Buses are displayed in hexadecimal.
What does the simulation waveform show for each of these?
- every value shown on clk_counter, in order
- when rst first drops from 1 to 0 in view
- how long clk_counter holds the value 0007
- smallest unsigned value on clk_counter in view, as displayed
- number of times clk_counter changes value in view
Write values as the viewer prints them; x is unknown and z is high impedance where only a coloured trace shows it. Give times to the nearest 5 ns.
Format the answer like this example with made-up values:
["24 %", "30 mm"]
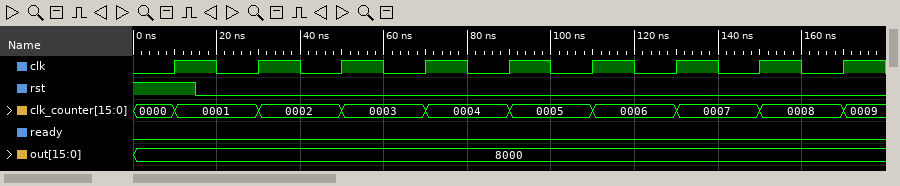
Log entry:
["0000, 0001, 0002, 0003, 0004, 0005, 0006, 0007, 0008, 0009", "15 ns", "20 ns", "0000", "9"]
